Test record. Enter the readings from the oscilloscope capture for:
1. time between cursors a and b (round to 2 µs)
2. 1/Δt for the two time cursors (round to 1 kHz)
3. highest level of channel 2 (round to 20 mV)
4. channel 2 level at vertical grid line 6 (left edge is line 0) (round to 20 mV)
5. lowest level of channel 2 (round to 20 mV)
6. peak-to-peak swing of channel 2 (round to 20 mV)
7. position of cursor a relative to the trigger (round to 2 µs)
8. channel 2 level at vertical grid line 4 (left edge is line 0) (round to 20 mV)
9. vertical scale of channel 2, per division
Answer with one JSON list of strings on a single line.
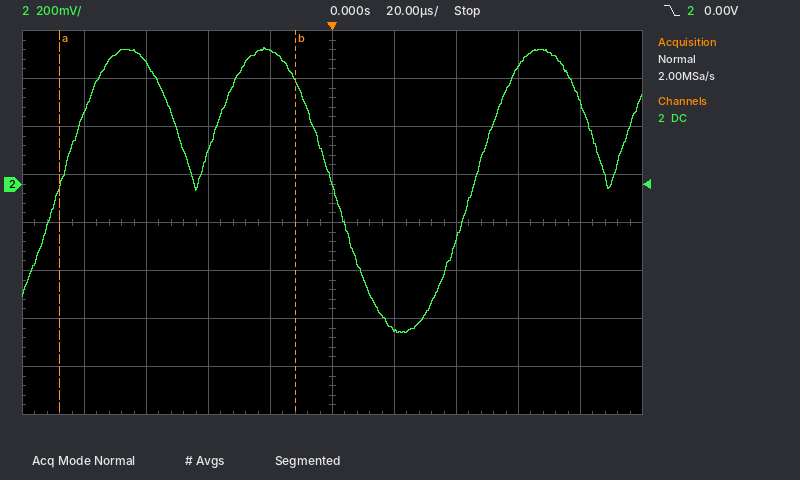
["76 µs", "13 kHz", "560 mV", "-600 mV", "-620 mV", "1.18 V", "-88 µs", "560 mV", "200 mV"]
